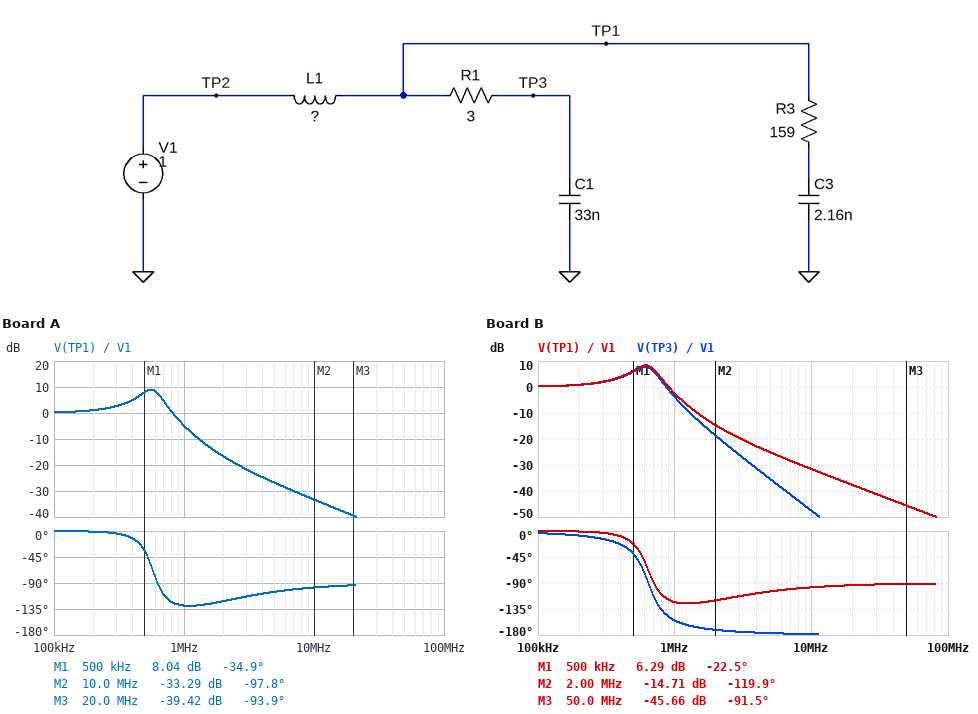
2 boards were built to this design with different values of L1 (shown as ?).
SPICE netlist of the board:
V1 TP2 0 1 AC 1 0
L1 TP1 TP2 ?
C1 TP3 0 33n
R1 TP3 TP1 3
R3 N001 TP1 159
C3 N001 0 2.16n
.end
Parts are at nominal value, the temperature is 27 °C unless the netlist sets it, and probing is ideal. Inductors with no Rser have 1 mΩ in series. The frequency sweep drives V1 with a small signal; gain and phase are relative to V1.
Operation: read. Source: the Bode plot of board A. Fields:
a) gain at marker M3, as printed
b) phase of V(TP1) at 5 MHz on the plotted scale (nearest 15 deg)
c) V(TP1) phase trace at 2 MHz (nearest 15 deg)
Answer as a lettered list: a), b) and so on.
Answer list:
a) -39.42 dB
b) -105 deg
c) -120 deg
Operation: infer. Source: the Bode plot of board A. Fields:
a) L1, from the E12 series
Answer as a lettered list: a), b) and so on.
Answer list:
a) 2.2 µH
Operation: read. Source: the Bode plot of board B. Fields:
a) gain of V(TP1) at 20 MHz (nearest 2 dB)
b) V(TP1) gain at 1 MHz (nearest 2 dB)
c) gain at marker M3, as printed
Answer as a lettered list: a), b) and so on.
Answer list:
a) -38 dB
b) -2 dB
c) -45.66 dB
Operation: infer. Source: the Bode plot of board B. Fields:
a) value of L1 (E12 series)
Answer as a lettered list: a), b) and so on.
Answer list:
a) 1.8 µH
